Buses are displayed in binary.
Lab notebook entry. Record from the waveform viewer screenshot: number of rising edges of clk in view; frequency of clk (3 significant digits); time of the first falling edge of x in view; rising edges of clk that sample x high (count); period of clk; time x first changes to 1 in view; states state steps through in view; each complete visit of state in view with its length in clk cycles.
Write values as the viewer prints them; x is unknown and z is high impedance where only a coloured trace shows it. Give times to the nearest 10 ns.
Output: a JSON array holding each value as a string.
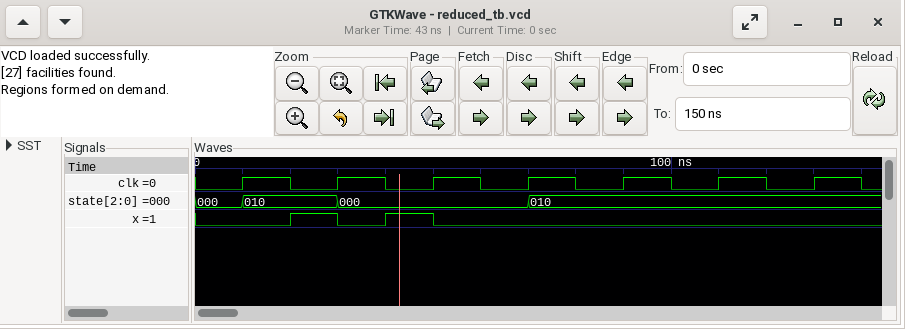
["7", "50.0 MHz", "30 ns", "2", "20 ns", "20 ns", "000, 010, 000, 010", "010: 1, 000: 2"]
